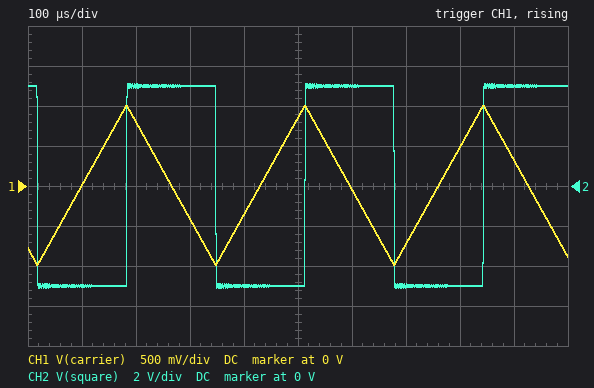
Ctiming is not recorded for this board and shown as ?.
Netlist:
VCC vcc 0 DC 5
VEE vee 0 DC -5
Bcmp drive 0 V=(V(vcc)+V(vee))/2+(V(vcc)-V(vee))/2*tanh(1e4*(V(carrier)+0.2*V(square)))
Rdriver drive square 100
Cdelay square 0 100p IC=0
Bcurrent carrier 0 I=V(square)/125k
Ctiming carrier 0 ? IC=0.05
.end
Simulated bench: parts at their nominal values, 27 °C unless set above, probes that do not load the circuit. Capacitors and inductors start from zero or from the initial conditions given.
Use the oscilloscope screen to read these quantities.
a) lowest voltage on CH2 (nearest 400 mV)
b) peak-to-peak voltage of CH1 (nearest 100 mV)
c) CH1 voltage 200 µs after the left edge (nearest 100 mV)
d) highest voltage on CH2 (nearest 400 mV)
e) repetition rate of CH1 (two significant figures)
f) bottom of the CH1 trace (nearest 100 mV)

-5.2 V
2.0 V
800 mV
5.2 V
3.0 kHz
-1.0 V
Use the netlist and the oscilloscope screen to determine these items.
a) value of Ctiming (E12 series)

3.3 nF
